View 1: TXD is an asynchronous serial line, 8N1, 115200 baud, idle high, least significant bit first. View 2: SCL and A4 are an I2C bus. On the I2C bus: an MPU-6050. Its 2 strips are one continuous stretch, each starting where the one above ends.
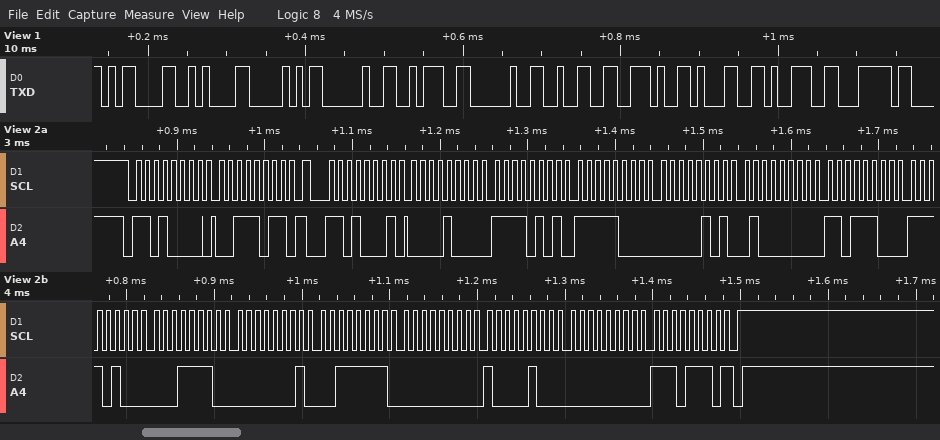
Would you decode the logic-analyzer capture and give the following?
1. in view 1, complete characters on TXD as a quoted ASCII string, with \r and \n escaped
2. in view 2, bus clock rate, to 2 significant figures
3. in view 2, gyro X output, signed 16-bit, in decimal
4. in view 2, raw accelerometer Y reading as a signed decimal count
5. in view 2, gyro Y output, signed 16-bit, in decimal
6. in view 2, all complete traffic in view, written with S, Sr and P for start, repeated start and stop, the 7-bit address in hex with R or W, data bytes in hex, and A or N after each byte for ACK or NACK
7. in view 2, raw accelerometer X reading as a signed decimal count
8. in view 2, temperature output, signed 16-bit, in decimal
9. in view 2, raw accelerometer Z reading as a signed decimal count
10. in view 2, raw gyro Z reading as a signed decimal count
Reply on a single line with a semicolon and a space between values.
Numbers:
"\r\nP : 2.19|"; 100 kHz; 319; -2043; 132; S 68W A 3B A Sr 68R A 08 A F5 A F8 A 05 A 40 A DC A F4 A 1E A 01 A 3F A 00 A 84 A 00 A EE N P; 2293; -3042; 16604; 238
